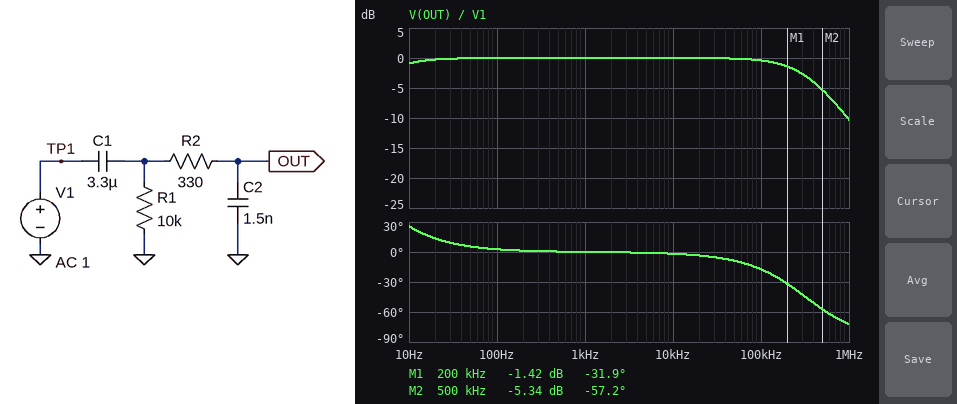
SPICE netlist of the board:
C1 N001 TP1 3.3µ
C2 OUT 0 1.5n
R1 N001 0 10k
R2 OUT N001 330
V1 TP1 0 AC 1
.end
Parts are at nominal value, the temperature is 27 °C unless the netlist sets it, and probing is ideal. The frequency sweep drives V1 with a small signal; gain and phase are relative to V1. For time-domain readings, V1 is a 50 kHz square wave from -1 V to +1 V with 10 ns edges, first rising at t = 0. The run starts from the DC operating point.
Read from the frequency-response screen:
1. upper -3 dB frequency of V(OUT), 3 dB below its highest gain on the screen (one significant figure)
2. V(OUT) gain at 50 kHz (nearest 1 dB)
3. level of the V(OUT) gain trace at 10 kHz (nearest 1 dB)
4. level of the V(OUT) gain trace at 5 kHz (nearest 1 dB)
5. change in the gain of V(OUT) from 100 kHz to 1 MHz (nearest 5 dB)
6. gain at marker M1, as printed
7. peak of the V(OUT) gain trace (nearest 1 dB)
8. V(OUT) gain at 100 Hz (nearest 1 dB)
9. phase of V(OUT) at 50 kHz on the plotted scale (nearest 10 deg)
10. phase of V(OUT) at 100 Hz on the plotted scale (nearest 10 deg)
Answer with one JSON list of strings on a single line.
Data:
["300 kHz", "0 dB", "0 dB", "0 dB", "-10 dB", "-1.42 dB", "0 dB", "0 dB", "-10 deg", "0 deg"]
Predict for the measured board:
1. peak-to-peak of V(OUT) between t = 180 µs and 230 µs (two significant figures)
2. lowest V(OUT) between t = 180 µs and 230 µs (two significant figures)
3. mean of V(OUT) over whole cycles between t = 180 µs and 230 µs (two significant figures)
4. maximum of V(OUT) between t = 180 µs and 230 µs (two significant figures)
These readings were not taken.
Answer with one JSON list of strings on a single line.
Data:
["2.0 V", "-6.6 mV", "990 mV", "2.0 V"]
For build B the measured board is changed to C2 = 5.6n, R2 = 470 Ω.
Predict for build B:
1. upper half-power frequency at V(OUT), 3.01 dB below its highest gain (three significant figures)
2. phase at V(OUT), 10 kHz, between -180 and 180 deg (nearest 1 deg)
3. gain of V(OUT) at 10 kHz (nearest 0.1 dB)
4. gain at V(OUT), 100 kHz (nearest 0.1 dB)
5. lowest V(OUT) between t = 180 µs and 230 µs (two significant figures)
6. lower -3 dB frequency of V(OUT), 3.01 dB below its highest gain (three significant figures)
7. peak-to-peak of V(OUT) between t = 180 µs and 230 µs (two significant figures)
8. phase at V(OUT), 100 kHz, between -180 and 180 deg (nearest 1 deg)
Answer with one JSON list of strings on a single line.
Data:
["60.6 kHz", "-9 deg", "-0.1 dB", "-5.7 dB", "37 mV", "4.81 Hz", "1.9 V", "-59 deg"]
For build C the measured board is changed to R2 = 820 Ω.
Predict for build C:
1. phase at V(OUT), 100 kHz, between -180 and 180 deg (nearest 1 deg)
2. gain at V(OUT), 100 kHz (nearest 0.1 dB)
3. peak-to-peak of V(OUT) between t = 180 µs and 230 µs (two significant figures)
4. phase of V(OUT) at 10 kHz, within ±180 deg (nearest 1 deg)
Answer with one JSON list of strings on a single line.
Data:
["-38 deg", "-2.0 dB", "2.0 V", "-4 deg"]
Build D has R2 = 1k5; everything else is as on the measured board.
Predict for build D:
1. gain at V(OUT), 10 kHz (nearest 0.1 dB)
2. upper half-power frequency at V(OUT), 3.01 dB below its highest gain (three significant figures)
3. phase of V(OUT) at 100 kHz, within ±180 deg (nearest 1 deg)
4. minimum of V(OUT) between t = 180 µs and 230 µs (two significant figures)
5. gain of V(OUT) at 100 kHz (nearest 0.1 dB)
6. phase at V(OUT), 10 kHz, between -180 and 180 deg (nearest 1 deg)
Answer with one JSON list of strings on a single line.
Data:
["-0.1 dB", "70.8 kHz", "-55 deg", "17 mV", "-4.8 dB", "-8 deg"]
